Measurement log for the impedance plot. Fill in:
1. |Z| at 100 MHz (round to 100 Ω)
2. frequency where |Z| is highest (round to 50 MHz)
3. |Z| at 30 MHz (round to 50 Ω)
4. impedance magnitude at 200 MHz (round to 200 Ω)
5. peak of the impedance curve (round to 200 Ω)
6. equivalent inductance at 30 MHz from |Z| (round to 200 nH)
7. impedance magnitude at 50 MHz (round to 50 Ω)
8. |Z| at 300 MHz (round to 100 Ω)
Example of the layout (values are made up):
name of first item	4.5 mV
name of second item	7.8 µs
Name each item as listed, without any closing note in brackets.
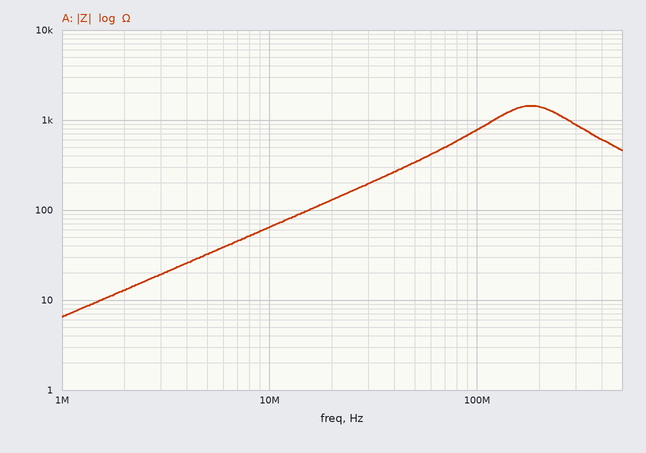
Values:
|Z| at 100 MHz	800 Ω
frequency where |Z| is highest	200 MHz
|Z| at 30 MHz	200 Ω
impedance magnitude at 200 MHz	1.4 kΩ
peak of the impedance curve	1.4 kΩ
equivalent inductance at 30 MHz from |Z|	1.0 µH
impedance magnitude at 50 MHz	350 Ω
|Z| at 300 MHz	900 Ω
